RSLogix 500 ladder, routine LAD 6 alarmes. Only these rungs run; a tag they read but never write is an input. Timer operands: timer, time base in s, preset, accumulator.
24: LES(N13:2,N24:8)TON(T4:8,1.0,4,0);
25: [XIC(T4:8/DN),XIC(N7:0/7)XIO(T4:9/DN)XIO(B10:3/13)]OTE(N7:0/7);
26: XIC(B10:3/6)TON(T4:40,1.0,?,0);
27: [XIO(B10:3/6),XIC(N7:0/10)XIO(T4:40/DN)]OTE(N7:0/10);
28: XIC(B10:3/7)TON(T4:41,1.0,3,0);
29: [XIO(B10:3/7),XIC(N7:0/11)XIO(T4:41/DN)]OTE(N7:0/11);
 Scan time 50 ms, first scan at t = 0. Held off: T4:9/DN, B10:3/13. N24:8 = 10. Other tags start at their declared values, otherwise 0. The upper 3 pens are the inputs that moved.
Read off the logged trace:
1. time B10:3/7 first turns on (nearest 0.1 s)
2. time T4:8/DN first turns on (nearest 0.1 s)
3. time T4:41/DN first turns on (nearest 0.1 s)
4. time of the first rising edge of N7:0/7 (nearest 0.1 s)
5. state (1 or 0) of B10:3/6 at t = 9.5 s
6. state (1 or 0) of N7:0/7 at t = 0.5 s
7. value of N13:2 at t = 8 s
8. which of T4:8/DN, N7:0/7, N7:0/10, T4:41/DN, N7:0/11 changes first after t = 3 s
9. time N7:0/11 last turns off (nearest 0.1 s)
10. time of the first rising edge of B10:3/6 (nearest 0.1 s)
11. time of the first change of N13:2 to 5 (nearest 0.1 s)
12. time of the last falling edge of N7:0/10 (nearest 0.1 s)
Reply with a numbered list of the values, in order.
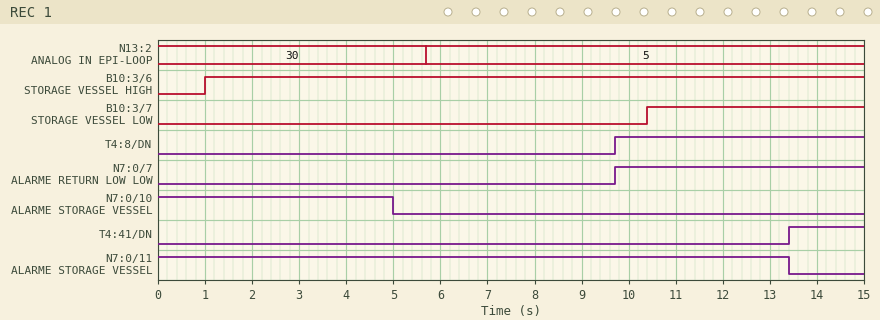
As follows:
1. 10.4 s
2. 9.7 s
3. 13.4 s
4. 9.7 s
5. 1
6. 0
7. 5
8. N7:0/10
9. 13.4 s
10. 1.0 s
11. 5.7 s
12. 5.0 s
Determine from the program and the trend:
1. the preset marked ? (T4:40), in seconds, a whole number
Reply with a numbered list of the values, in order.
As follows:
1. 4 s
